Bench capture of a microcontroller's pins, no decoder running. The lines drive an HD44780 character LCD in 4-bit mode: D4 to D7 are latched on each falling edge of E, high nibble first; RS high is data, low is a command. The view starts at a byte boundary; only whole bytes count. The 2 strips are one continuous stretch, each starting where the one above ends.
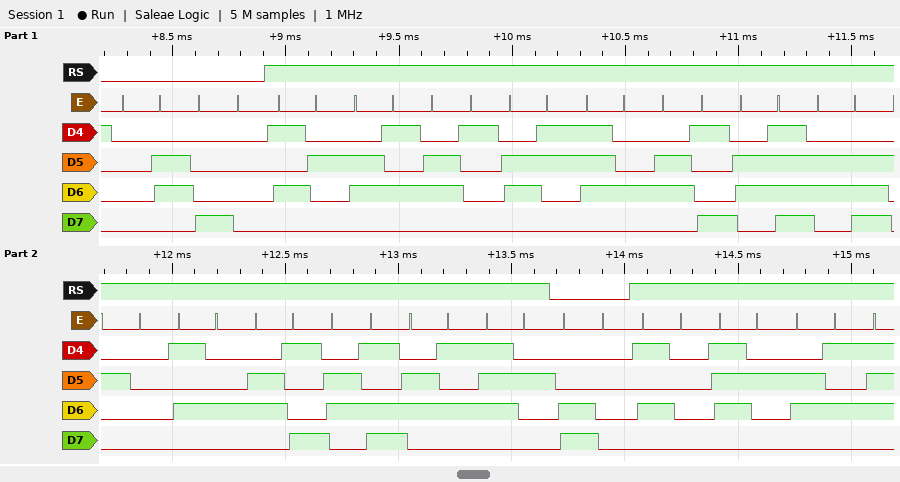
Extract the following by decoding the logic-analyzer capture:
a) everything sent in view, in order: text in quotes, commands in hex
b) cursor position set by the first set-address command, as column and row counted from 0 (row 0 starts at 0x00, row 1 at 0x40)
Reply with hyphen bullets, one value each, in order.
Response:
- 0x06 0x80 "Reaction Timer" 0xC0 "Pre"
- column 0, row 0
